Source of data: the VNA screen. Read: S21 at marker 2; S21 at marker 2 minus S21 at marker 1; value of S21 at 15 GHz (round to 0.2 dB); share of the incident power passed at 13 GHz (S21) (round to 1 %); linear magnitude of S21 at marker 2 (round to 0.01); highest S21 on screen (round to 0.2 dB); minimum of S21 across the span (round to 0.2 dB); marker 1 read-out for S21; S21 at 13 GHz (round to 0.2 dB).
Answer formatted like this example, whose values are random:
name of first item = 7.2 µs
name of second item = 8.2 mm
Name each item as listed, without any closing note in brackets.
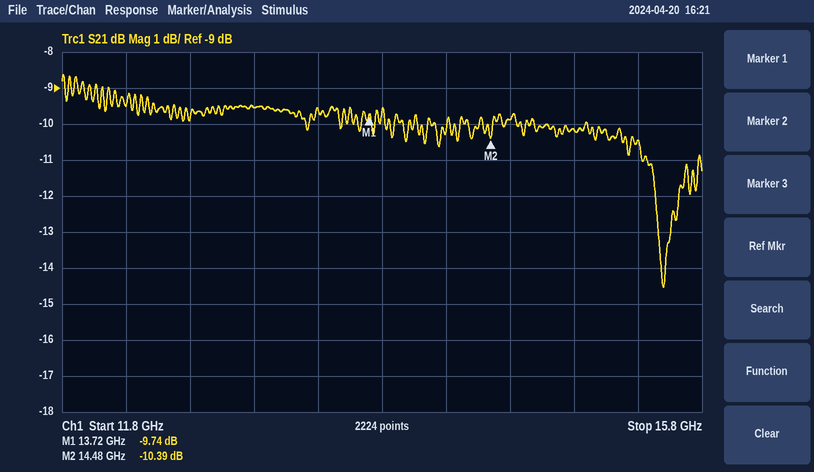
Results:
S21 at marker 2 = -10.39 dB
S21 at marker 2 minus S21 at marker 1 = -0.65 dB
value of S21 at 15 GHz = -10.2 dB
share of the incident power passed at 13 GHz (S21) = 11 %
linear magnitude of S21 at marker 2 = 0.30
highest S21 on screen = -8.6 dB
minimum of S21 across the span = -14.6 dB
marker 1 read-out for S21 = -9.74 dB
S21 at 13 GHz = -9.6 dB
